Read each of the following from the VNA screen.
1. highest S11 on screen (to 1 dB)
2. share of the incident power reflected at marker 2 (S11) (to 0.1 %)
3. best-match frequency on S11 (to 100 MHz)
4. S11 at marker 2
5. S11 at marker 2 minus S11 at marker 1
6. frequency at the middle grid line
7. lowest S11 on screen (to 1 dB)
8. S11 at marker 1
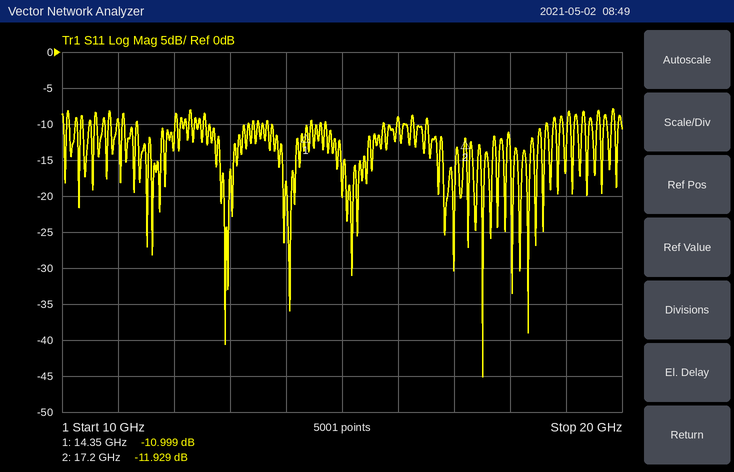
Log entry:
-8 dB
6.4 %
17.5 GHz
-11.929 dB
-0.930 dB
15 GHz
-45 dB
-10.999 dB
